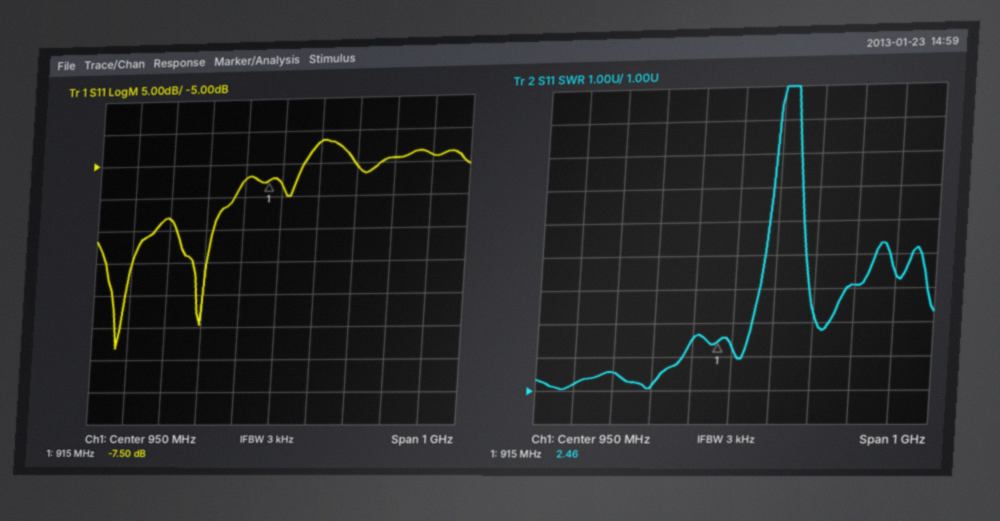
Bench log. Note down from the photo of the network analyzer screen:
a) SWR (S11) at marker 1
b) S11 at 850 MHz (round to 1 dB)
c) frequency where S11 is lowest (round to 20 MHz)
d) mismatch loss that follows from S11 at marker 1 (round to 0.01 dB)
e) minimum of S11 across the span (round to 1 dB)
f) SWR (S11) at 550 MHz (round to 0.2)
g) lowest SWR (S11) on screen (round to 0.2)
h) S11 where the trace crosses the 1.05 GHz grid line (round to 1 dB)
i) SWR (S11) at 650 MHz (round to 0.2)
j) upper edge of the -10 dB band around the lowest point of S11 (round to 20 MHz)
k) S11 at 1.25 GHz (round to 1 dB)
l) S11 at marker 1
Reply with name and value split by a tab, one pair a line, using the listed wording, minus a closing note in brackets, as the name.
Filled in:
SWR (S11) at marker 1	2.46
S11 at 850 MHz	-7 dB
frequency where S11 is lowest	520 MHz
mismatch loss that follows from S11 at marker 1	0.85 dB
minimum of S11 across the span	-33 dB
SWR (S11) at 550 MHz	1.2
lowest SWR (S11) on screen	1.0
S11 where the trace crosses the 1.05 GHz grid line	-2 dB
SWR (S11) at 650 MHz	1.6
upper edge of the -10 dB band around the lowest point of S11	820 MHz
S11 at 1.25 GHz	-4 dB
S11 at marker 1	-7.50 dB
